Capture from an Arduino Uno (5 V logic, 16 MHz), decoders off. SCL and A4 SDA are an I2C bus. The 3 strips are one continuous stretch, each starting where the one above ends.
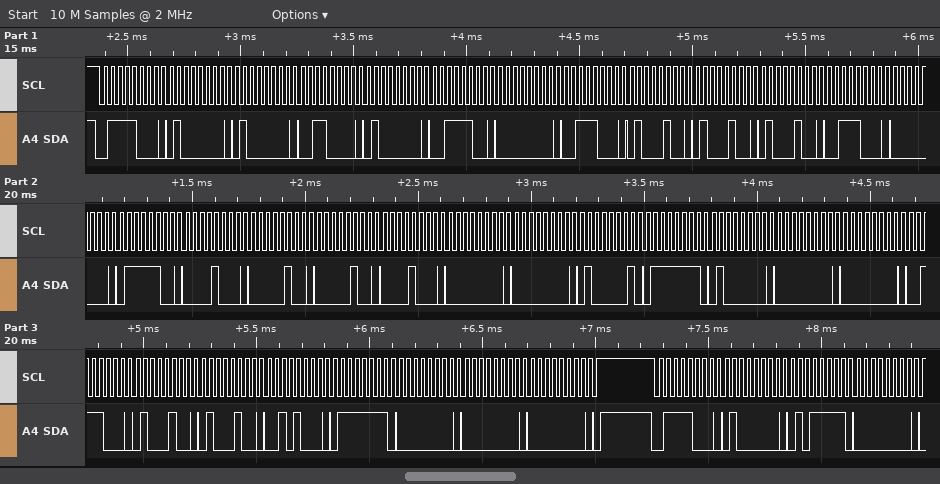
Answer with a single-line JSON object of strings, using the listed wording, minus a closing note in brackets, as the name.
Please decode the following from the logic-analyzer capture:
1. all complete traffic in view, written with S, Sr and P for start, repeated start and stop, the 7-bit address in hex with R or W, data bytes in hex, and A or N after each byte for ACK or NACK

{"all complete traffic in view, written with S, Sr and P for start, repeated start and stop, the 7-bit address in hex with R or W, data bytes in hex, and A or N after each byte for ACK or NACK": "S 3CW A 40 A 40 A 30 A 40 A 3C A 00 A 38 A 44 A 44 A 44 A 38 A 00 A 7C A 08 A 04 A 04 A 08 A 00 A 00 A 41 A 7F A 40 A 00 A 00 A 38 A 44 A 44 A 28 A 7F A 00 A 00 A 00 A P S 3CW A 40 A 5F A 00 A"}
